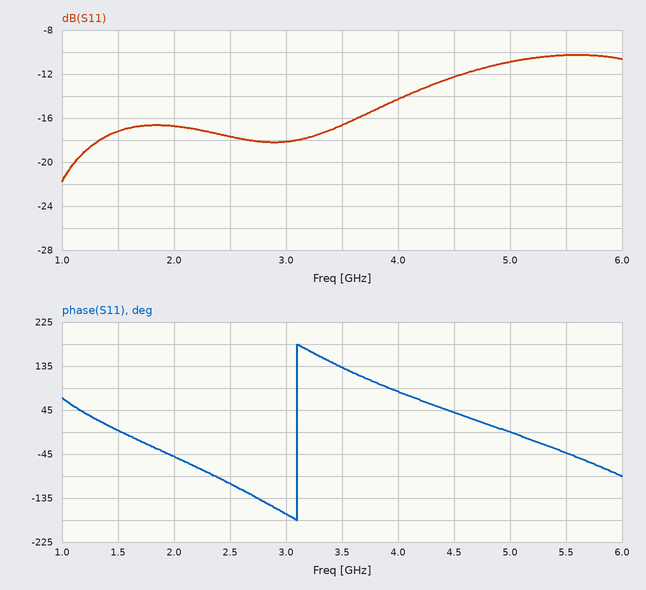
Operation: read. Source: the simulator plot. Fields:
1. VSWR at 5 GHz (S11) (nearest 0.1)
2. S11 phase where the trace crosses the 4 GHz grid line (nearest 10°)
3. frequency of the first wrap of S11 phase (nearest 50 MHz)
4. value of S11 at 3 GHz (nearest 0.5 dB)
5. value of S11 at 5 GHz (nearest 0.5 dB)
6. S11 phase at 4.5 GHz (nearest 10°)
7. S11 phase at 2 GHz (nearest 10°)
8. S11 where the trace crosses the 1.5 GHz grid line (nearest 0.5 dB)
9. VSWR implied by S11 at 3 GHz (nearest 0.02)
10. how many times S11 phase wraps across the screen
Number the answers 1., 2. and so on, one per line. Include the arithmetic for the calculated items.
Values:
1. |Γ| = 10^(-11/20) = 0.2818; VSWR = (1 + 0.2818)/(1 − 0.2818) ≈ 1.8
2. 80°
3. 3.10 GHz
4. -18.0 dB
5. -11.0 dB
6. 40°
7. -50°
8. -17.0 dB
9. |Γ| = 10^(-18/20) = 0.1259; VSWR = (1 + 0.1259)/(1 − 0.1259) ≈ 1.29, so 1.28 to the nearest 0.02
10. 1
